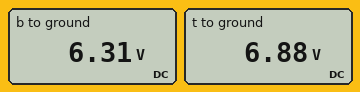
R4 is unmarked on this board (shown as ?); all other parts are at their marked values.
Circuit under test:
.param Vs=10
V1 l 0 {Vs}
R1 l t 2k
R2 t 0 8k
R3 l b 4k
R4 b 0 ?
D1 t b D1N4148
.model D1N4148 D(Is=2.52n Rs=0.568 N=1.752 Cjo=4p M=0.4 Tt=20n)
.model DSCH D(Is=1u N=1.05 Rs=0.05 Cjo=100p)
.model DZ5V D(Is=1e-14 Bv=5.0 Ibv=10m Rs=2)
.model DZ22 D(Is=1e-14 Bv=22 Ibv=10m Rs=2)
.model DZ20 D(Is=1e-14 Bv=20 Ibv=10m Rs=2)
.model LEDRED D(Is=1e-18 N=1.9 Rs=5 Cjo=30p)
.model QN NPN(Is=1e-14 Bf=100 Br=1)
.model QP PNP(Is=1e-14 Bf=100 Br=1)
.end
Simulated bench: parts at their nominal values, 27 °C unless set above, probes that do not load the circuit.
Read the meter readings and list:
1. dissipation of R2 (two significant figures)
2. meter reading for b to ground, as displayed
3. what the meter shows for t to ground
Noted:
5.9 mW
6.31 V
6.88 V
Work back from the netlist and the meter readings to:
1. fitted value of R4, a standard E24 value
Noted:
3.9 kΩ
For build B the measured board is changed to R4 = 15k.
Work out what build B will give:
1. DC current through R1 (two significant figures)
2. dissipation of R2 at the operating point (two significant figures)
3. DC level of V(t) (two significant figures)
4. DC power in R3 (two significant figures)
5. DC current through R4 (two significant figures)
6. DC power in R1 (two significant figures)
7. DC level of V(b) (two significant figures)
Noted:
1.0 mA
8.0 mW
8.0 V
1.1 mW
530 µA
2.0 mW
7.9 V
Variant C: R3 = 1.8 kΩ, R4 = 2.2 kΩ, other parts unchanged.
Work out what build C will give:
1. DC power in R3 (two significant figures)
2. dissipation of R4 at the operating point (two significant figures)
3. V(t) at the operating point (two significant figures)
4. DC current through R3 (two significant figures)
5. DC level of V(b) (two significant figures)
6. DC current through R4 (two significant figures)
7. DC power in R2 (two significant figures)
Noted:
7.9 mW
18 mW
6.8 V
2.1 mA
6.2 V
2.8 mA
5.8 mW
